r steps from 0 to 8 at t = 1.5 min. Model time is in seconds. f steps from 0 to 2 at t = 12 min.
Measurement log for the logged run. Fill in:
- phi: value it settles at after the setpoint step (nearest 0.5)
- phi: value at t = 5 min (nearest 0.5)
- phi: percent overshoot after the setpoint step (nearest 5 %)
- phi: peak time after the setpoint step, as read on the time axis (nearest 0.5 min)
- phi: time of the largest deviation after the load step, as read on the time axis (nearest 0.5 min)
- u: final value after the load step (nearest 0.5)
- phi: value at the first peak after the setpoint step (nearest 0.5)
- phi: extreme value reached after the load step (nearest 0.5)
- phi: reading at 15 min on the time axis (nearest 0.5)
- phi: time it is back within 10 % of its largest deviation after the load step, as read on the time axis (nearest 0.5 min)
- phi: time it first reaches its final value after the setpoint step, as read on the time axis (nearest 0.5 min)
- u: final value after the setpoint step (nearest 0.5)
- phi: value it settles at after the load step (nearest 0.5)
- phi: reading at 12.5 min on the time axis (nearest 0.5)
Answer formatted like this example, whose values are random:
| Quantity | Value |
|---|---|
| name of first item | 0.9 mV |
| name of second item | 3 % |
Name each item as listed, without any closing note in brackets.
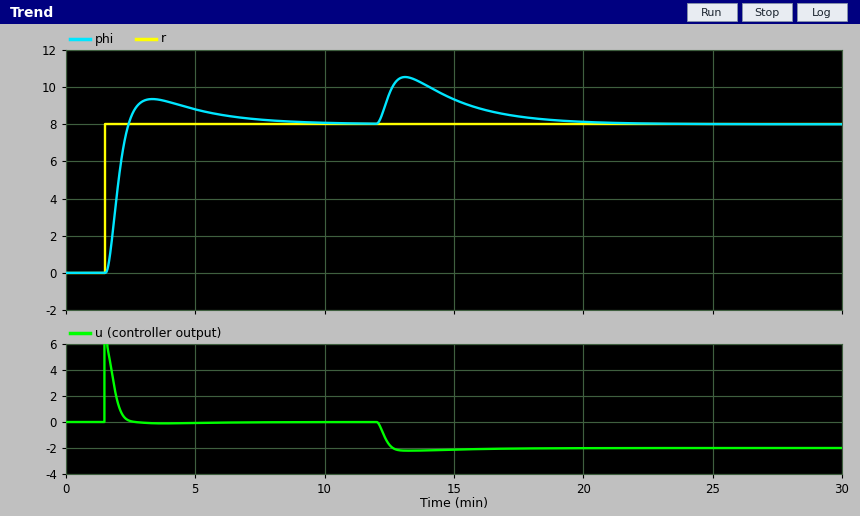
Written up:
| Quantity | Value |
|---|---|
| phi: value it settles at after the setpoint step | 8.0 |
| phi: value at t = 5 min | 9.0 |
| phi: percent overshoot after the setpoint step | 15 % |
| phi: peak time after the setpoint step, as read on the time axis | 3.5 min |
| phi: time of the largest deviation after the load step, as read on the time axis | 13.0 min |
| u: final value after the load step | -2.0 |
| phi: value at the first peak after the setpoint step | 9.5 |
| phi: extreme value reached after the load step | 10.5 |
| phi: reading at 15 min on the time axis | 9.5 |
| phi: time it is back within 10 % of its largest deviation after the load step, as read on the time axis | 18.5 min |
| phi: time it first reaches its final value after the setpoint step, as read on the time axis | 2.5 min |
| u: final value after the setpoint step | 0.0 |
| phi: value it settles at after the load step | 8.0 |
| phi: reading at 12.5 min on the time axis | 9.5 |
